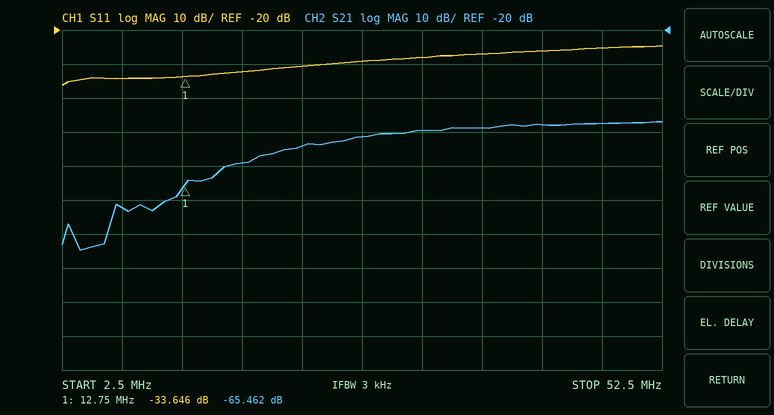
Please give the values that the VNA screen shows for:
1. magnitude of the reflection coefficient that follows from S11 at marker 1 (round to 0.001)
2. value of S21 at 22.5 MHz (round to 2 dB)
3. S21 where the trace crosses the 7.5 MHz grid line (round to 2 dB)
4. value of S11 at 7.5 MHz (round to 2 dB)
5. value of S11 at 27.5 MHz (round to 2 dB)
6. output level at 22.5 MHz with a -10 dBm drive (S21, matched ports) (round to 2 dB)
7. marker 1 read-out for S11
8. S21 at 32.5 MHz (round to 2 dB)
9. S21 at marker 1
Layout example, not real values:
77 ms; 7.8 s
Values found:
0.021; -54 dB; -72 dB; -34 dB; -30 dB; -64 dBm; -33.646 dB; -50 dB; -65.462 dB
